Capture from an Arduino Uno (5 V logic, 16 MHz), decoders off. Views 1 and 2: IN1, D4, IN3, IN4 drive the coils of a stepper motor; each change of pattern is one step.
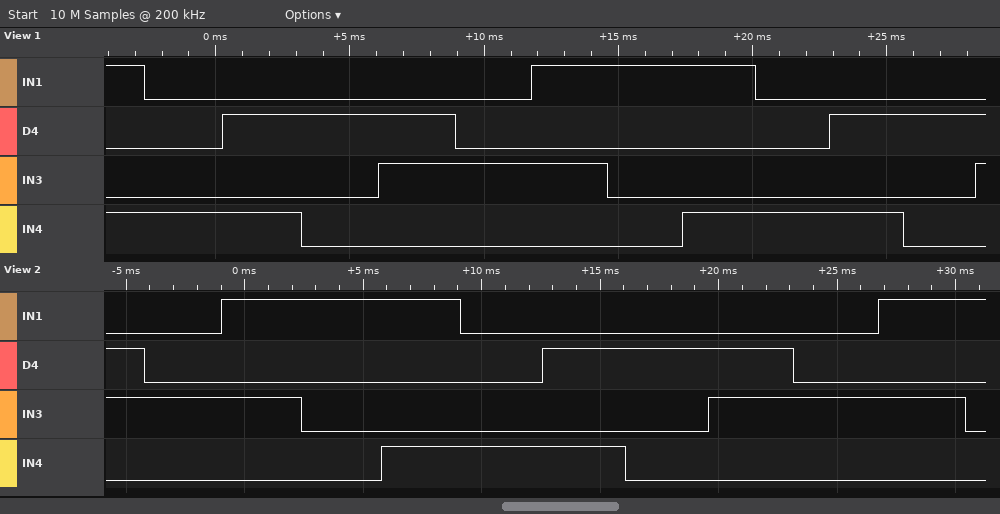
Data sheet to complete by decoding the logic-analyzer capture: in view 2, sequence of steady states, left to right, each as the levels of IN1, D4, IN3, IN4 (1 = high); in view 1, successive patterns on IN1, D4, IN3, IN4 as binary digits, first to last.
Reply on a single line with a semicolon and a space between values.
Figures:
0110 0010 1010 1000 1001 0001 0101 0100 0110 0010 1010 1000; 1001 0001 0101 0100 0110 0010 1010 1000 1001 0001 0101 0100 0110
